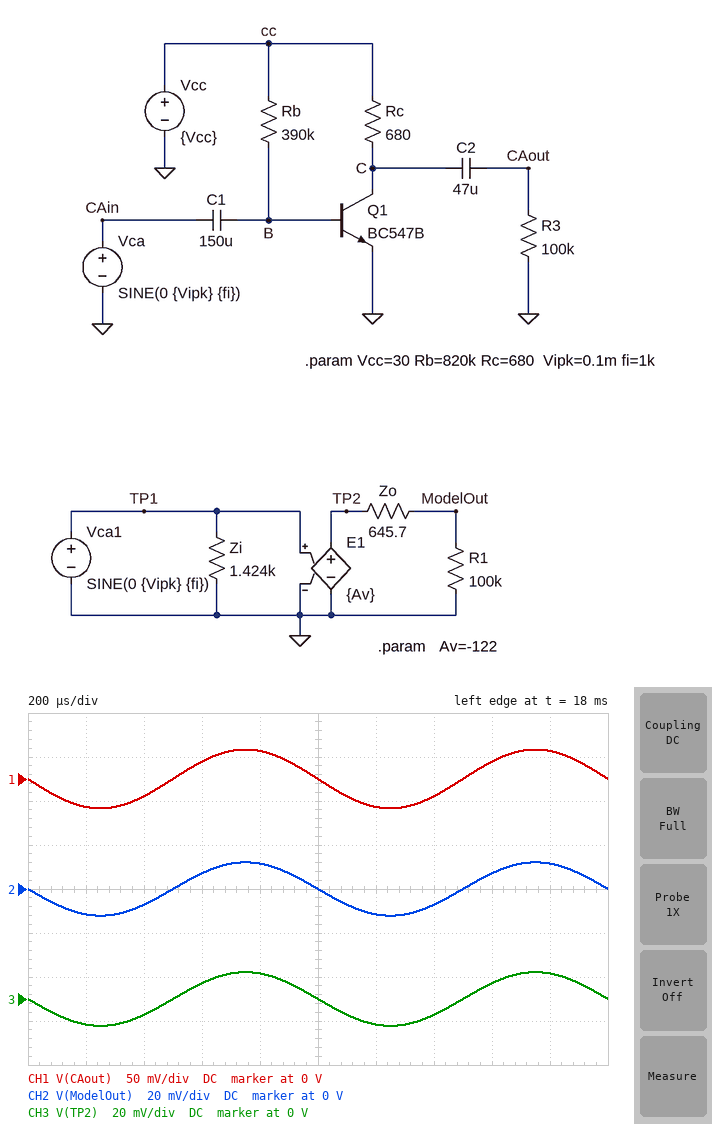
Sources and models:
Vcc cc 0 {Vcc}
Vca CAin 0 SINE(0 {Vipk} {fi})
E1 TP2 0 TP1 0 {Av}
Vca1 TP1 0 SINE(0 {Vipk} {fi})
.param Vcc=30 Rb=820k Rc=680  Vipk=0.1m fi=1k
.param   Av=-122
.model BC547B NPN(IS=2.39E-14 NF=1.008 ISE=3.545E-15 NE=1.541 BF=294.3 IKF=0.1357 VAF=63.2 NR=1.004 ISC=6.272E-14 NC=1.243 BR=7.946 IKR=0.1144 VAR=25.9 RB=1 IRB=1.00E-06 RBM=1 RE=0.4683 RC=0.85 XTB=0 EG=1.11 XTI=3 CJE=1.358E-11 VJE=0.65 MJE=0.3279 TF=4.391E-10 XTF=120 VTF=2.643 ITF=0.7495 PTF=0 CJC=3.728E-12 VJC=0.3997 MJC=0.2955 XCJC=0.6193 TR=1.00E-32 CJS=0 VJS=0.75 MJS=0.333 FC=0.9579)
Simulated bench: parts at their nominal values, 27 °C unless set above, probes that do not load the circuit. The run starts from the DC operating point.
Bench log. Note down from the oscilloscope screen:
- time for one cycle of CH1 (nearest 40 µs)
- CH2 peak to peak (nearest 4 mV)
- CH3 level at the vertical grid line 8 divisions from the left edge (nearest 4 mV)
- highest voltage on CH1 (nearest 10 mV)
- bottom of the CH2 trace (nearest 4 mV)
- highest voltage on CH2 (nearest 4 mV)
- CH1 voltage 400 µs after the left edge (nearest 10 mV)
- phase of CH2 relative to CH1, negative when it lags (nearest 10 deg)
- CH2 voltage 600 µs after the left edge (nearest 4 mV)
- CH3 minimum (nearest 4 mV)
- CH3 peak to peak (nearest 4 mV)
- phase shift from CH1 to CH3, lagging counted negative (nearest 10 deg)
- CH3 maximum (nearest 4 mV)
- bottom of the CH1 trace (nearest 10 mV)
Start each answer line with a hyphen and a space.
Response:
- 1.00 ms
- 24 mV
- 8 mV
- 30 mV
- -12 mV
- 12 mV
- -20 mV
- 0 deg
- 8 mV
- -12 mV
- 24 mV
- 0 deg
- 12 mV
- -30 mV
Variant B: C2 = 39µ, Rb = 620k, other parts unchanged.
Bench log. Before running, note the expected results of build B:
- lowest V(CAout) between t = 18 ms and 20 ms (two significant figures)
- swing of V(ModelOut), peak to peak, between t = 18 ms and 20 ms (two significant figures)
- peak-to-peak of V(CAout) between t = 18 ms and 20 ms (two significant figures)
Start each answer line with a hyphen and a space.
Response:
- -27 mV
- 24 mV
- 54 mV
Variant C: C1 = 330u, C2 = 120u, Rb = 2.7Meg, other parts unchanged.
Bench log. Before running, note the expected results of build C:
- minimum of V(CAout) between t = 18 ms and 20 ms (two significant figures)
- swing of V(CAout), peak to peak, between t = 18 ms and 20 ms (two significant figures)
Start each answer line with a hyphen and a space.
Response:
- -9.9 mV
- 20 mV
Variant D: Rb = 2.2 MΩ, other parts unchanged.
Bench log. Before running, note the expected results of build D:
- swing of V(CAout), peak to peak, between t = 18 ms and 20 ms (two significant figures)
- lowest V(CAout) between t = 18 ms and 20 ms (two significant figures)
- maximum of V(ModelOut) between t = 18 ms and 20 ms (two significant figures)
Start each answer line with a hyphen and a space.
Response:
- 23 mV
- -12 mV
- 12 mV
